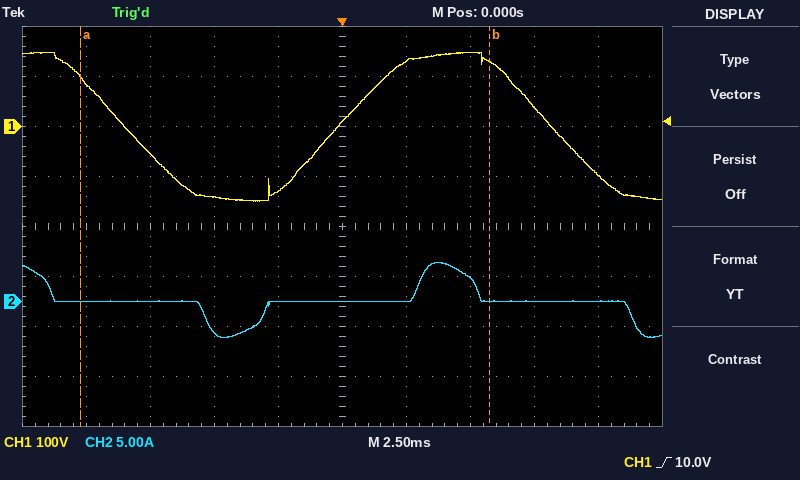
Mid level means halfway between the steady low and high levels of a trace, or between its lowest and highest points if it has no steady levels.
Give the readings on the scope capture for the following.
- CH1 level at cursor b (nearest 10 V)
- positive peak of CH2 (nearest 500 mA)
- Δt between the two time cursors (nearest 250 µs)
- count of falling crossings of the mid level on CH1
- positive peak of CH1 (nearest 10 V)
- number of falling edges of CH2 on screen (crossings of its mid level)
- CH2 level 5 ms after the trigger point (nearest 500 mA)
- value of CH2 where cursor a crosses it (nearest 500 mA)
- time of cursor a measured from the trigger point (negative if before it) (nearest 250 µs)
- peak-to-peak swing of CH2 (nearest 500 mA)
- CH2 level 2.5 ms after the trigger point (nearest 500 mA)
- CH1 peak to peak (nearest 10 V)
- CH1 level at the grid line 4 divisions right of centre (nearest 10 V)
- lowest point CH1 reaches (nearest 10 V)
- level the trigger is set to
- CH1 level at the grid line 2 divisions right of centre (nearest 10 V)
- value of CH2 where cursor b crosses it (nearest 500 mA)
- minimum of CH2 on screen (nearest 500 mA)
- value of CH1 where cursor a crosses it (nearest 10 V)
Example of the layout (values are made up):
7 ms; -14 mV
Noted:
130 V; 4.0 A; 16.00 ms; 2; 150 V; 2; 2.5 A; 0.0 A; -10.25 ms; 7.5 A; 0.0 A; 300 V; -100 V; -150 V; 10.0 V; 150 V; 0.0 A; -3.5 A; 100 V
